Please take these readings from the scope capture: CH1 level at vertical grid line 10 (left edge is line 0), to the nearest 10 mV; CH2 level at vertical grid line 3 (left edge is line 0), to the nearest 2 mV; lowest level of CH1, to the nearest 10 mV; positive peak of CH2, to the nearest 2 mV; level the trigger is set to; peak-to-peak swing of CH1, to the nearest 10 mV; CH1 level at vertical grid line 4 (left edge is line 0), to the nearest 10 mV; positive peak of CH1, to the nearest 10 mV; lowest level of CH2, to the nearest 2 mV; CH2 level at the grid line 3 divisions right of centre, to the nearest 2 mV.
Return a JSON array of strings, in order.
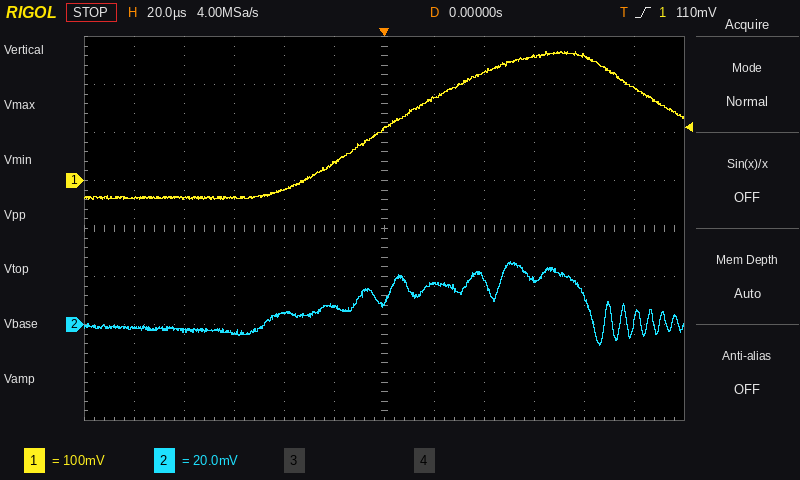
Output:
["260 mV", "-4 mV", "-40 mV", "26 mV", "110 mV", "310 mV", "-20 mV", "270 mV", "-8 mV", "18 mV"]
